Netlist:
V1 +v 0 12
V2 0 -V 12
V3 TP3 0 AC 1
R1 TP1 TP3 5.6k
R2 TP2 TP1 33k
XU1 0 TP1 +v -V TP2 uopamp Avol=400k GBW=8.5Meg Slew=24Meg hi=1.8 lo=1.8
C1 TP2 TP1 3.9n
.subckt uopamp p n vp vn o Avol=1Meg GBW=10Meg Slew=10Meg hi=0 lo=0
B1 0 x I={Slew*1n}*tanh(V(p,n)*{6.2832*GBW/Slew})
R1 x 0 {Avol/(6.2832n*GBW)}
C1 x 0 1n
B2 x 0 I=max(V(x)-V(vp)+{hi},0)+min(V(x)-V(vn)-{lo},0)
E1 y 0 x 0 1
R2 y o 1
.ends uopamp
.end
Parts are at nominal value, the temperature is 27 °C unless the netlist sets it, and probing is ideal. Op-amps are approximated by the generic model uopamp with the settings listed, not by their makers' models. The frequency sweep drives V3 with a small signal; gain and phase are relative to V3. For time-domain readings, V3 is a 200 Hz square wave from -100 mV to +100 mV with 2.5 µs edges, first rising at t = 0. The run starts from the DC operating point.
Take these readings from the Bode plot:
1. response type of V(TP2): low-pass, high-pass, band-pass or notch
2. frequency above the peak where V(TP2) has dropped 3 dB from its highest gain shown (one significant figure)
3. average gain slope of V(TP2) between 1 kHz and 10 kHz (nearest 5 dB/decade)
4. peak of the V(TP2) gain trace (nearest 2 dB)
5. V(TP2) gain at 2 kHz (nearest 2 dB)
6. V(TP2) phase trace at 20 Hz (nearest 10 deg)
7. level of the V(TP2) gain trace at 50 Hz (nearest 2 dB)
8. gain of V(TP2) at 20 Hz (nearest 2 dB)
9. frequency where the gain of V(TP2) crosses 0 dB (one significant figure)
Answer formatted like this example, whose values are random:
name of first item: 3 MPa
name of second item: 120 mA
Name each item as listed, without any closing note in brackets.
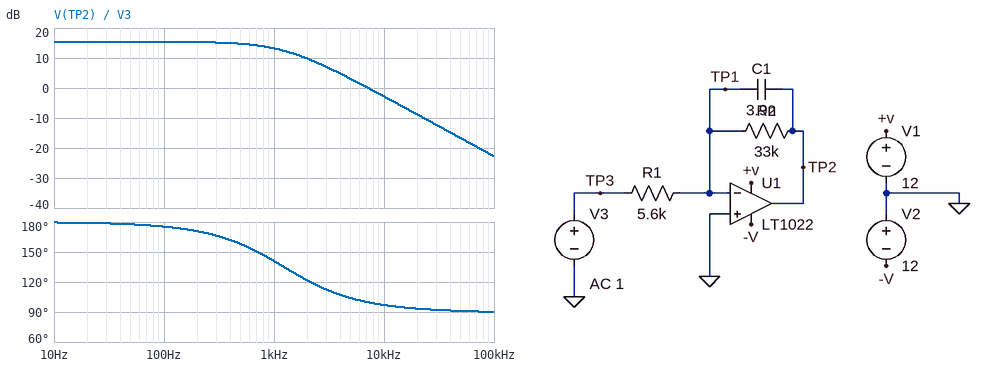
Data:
response type of V(TP2): low-pass, high-pass, band-pass or notch: low-pass
frequency above the peak where V(TP2) has dropped 3 dB from its highest gain shown: 1 kHz
average gain slope of V(TP2) between 1 kHz and 10 kHz: -15 dB/decade
peak of the V(TP2) gain trace: 16 dB
V(TP2) gain at 2 kHz: 10 dB
V(TP2) phase trace at 20 Hz: 180 deg
level of the V(TP2) gain trace at 50 Hz: 16 dB
gain of V(TP2) at 20 Hz: 16 dB
frequency where the gain of V(TP2) crosses 0 dB: 7 kHz
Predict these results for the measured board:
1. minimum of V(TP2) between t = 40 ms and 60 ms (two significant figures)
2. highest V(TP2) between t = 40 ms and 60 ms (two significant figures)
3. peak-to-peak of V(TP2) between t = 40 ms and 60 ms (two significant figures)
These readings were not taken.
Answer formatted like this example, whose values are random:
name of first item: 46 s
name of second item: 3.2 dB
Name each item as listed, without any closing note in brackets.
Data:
minimum of V(TP2) between t = 40 ms and 60 ms: -590 mV
highest V(TP2) between t = 40 ms and 60 ms: 590 mV
peak-to-peak of V(TP2) between t = 40 ms and 60 ms: 1.2 V
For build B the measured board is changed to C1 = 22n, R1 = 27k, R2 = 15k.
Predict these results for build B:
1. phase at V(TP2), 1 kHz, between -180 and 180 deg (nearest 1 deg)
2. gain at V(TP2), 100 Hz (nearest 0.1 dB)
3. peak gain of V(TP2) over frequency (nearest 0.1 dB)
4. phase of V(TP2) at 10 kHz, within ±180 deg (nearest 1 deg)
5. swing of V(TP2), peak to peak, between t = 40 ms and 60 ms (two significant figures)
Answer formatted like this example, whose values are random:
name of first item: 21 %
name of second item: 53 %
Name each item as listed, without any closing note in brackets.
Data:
phase at V(TP2), 1 kHz, between -180 and 180 deg: 116 deg
gain at V(TP2), 100 Hz: -5.3 dB
peak gain of V(TP2) over frequency: -5.1 dB
phase of V(TP2) at 10 kHz, within ±180 deg: 93 deg
swing of V(TP2), peak to peak, between t = 40 ms and 60 ms: 110 mV
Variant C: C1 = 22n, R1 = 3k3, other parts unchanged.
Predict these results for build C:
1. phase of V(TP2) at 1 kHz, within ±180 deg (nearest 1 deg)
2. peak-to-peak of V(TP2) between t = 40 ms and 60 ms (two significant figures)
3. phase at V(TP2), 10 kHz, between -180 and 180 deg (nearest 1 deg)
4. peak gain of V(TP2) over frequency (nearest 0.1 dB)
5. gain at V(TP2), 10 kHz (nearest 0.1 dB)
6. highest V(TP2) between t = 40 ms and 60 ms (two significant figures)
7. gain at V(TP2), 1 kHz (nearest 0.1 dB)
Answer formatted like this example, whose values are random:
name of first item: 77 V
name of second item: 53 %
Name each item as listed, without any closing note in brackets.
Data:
phase of V(TP2) at 1 kHz, within ±180 deg: 102 deg
peak-to-peak of V(TP2) between t = 40 ms and 60 ms: 1.9 V
phase at V(TP2), 10 kHz, between -180 and 180 deg: 91 deg
peak gain of V(TP2) over frequency: 20.0 dB
gain at V(TP2), 10 kHz: -13.2 dB
highest V(TP2) between t = 40 ms and 60 ms: 940 mV
gain at V(TP2), 1 kHz: 6.6 dB
